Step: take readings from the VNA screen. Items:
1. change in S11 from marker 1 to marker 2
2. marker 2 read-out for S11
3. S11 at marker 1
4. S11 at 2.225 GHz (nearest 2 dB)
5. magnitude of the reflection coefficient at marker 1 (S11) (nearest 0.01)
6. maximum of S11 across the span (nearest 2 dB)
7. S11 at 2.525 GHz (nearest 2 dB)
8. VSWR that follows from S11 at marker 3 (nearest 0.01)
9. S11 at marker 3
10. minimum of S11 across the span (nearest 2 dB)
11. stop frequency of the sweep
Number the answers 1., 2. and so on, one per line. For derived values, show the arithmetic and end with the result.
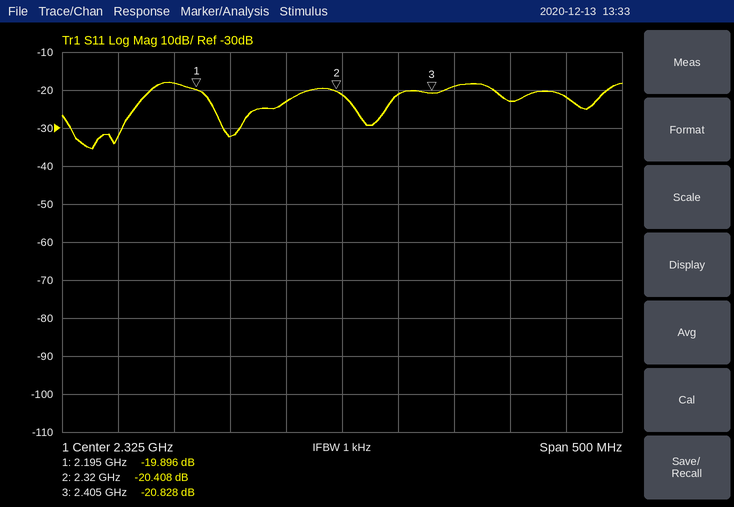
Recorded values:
1. -20.408 − (-19.896) = -0.512 dB
2. -20.408 dB
3. -19.896 dB
4. -32 dB
5. 10^(-19.896/20) ≈ 0.10
6. -18 dB
7. -22 dB
8. (1 + 0.0909)/(1 − 0.0909) ≈ 1.20
9. -20.828 dB
10. -36 dB
11. 2.575 GHz
